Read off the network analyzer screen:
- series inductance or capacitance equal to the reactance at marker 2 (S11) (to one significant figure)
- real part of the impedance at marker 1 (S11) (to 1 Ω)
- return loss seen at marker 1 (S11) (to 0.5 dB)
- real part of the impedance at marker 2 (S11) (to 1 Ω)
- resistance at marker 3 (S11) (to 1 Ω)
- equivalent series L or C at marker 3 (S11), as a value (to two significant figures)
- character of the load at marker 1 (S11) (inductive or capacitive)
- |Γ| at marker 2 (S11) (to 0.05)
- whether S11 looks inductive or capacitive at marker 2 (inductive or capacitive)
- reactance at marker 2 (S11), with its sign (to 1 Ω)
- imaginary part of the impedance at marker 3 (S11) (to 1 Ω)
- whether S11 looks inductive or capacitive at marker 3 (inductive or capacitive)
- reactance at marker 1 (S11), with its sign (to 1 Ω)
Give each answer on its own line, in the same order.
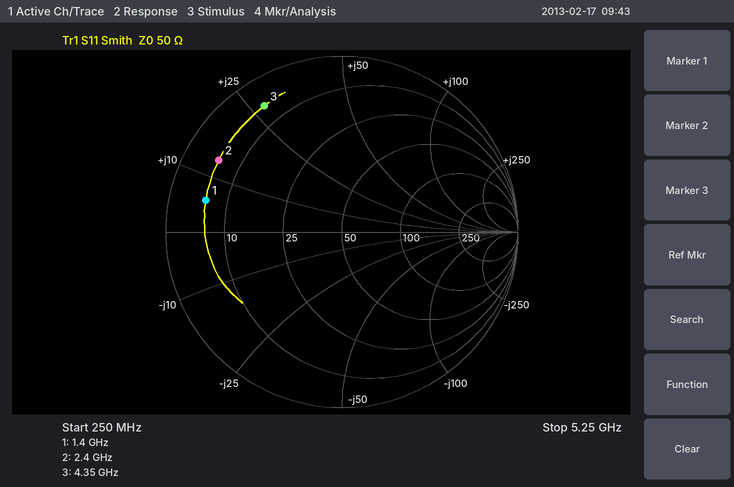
900 pH
6 Ω
2.0 dB
6 Ω
6 Ω
1.0 nH
inductive
0.80
inductive
+13 Ω
+28 Ω
inductive
+6 Ω
